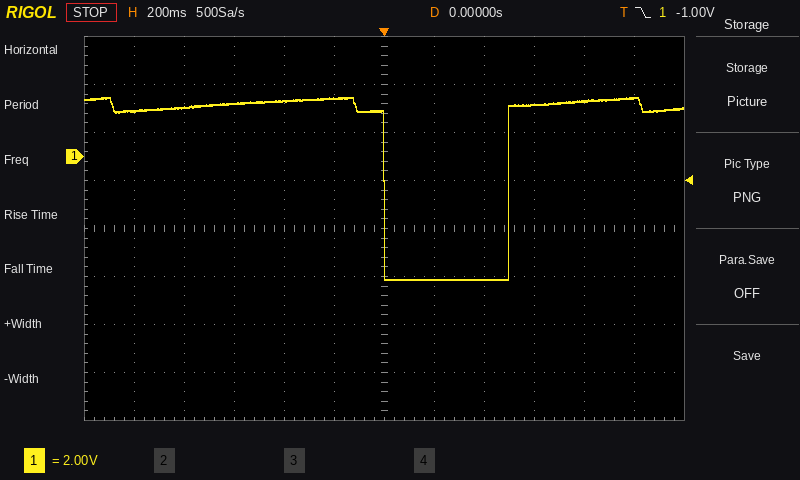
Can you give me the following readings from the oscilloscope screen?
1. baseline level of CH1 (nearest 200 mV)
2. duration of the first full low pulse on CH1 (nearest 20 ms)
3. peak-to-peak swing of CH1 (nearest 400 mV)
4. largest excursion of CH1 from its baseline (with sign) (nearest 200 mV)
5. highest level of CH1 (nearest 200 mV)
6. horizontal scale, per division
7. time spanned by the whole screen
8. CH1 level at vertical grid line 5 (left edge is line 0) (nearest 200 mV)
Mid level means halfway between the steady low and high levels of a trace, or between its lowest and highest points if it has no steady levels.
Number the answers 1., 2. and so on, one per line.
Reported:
1. 2.2 V
2. 500 ms
3. 7.6 V
4. -7.2 V
5. 2.4 V
6. 200 ms
7. 2.4 s
8. 2.4 V
